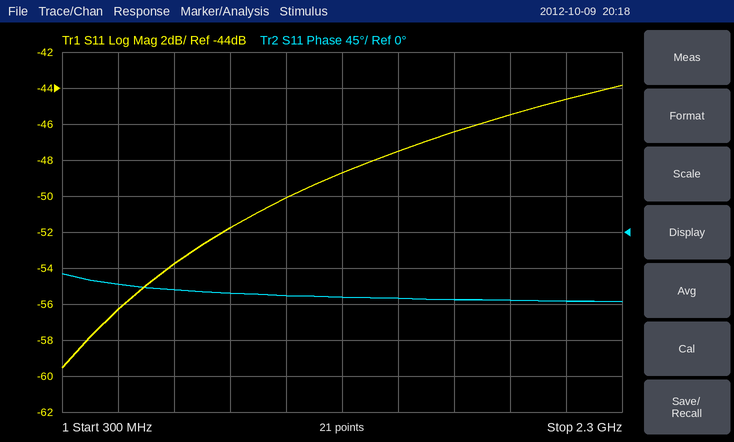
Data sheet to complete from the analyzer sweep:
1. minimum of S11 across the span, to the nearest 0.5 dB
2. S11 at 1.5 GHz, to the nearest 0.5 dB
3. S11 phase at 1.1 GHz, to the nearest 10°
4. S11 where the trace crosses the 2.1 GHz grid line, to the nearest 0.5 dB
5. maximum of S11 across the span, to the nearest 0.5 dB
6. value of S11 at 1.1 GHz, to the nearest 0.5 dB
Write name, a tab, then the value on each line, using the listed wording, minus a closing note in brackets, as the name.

minimum of S11 across the span, to the nearest 0.5 dB	-59.5 dB
S11 at 1.5 GHz, to the nearest 0.5 dB	-47.5 dB
S11 phase at 1.1 GHz, to the nearest 10°	-80°
S11 where the trace crosses the 2.1 GHz grid line, to the nearest 0.5 dB	-44.5 dB
maximum of S11 across the span, to the nearest 0.5 dB	-44.0 dB
value of S11 at 1.1 GHz, to the nearest 0.5 dB	-50.0 dB
